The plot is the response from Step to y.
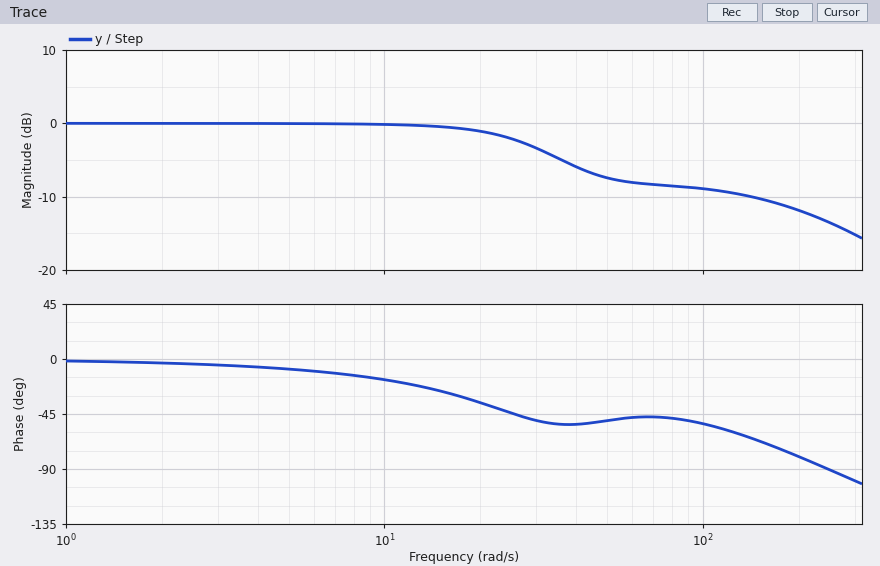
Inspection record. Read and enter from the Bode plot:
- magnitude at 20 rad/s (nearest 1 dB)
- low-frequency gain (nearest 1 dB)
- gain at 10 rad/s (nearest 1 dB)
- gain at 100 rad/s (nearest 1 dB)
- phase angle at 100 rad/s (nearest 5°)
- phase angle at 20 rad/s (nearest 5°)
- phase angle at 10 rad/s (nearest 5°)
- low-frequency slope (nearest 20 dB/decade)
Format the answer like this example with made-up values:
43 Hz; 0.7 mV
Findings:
-1 dB; 0 dB; 0 dB; -9 dB; -55°; -35°; -15°; 0 dB/decade
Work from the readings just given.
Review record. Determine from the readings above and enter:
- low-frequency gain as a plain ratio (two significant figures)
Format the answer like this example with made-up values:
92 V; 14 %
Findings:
1.0
